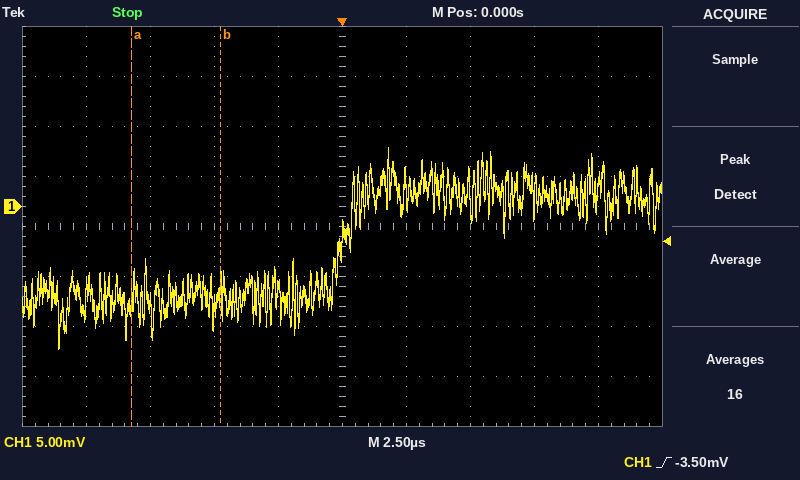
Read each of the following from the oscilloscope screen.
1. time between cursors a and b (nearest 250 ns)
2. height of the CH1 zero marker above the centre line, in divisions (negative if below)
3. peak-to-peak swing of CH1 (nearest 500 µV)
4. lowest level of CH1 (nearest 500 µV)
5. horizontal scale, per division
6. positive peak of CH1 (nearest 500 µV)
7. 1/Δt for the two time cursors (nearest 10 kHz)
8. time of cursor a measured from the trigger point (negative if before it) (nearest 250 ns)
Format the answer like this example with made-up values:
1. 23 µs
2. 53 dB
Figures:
1. 3.50 µs
2. +0.4 div
3. 20.0 mV
4. -14.0 mV
5. 2.5 µs
6. 6.0 mV
7. 290 kHz
8. -8.25 µs
